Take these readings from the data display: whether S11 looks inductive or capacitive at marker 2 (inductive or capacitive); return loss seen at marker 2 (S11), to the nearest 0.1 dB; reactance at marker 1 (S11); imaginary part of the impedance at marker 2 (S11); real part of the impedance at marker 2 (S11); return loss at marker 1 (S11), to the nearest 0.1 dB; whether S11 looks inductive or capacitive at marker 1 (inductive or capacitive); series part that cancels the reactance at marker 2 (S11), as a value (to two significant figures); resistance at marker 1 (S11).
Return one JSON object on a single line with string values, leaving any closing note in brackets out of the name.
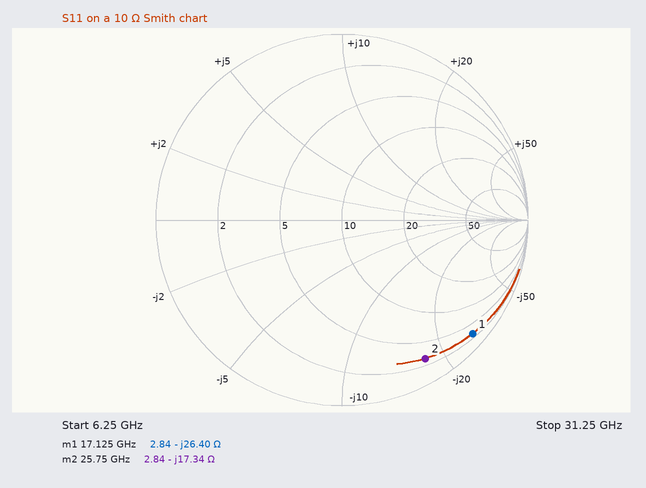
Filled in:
{"whether S11 looks inductive or capacitive at marker 2": "capacitive", "return loss seen at marker 2 (S11), to the nearest 0.1 dB": "1.2 dB", "reactance at marker 1": "-26.40 Ω", "imaginary part of the impedance at marker 2": "-17.34 Ω", "real part of the impedance at marker 2": "2.84 Ω", "return loss at marker 1 (S11), to the nearest 0.1 dB": "0.6 dB", "whether S11 looks inductive or capacitive at marker 1": "capacitive", "series part that cancels the reactance at marker 2 (S11), as a value": "110 pH", "resistance at marker 1": "2.84 Ω"}
